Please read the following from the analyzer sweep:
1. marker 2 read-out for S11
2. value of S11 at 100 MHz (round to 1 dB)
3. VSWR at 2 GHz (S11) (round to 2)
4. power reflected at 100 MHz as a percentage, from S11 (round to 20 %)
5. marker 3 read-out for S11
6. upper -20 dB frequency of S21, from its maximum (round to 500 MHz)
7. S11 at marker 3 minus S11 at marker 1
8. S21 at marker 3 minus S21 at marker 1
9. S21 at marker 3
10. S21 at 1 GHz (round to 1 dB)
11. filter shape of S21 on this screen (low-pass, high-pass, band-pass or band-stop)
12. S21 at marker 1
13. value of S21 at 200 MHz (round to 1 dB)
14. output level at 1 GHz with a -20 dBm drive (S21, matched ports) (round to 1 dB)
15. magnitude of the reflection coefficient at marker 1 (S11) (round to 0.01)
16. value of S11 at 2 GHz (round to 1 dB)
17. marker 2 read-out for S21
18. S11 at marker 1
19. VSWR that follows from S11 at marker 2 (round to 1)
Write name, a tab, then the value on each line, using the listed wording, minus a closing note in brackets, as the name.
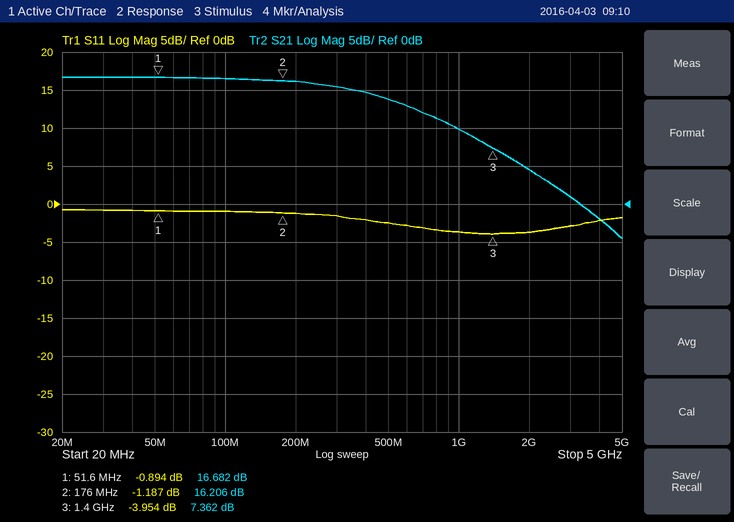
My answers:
marker 2 read-out for S11	-1.187 dB
value of S11 at 100 MHz	-1 dB
VSWR at 2 GHz (S11)	4
power reflected at 100 MHz as a percentage, from S11	80 %
marker 3 read-out for S11	-3.954 dB
upper -20 dB frequency of S21, from its maximum	4.5 GHz
S11 at marker 3 minus S11 at marker 1	-3.060 dB
S21 at marker 3 minus S21 at marker 1	-9.320 dB
S21 at marker 3	7.362 dB
S21 at 1 GHz	10 dB
filter shape of S21 on this screen	low-pass
S21 at marker 1	16.682 dB
value of S21 at 200 MHz	16 dB
output level at 1 GHz with a -20 dBm drive (S21, matched ports)	-10 dBm
magnitude of the reflection coefficient at marker 1 (S11)	0.90
value of S11 at 2 GHz	-4 dB
marker 2 read-out for S21	16.206 dB
S11 at marker 1	-0.894 dB
VSWR that follows from S11 at marker 2	15
